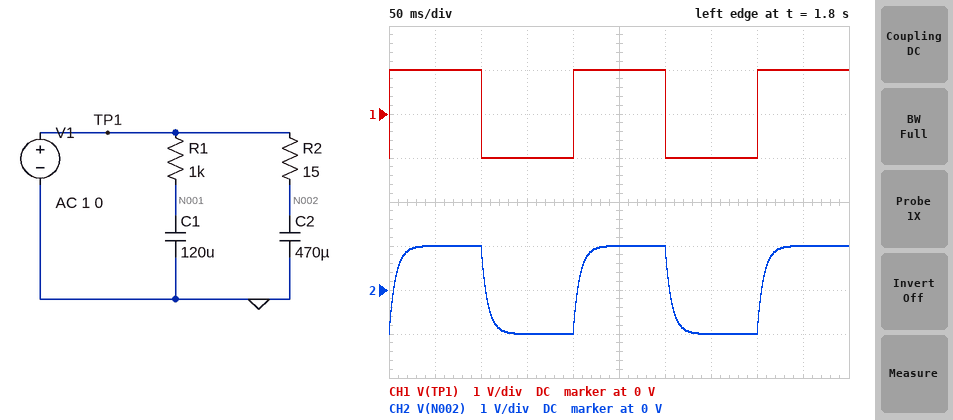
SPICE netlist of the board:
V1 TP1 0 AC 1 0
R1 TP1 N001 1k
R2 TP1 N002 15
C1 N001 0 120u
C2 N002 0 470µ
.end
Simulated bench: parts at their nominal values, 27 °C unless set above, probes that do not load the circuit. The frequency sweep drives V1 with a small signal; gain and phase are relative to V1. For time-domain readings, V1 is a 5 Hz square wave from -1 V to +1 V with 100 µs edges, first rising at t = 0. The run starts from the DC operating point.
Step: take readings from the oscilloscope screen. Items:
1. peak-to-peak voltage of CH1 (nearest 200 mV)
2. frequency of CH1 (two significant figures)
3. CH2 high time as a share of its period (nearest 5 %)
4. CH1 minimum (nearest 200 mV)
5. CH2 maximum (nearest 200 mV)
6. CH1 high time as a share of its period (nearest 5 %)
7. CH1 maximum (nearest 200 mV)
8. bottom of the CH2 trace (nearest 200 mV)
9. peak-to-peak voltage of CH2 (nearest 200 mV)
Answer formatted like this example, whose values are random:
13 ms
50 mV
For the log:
2.0 V
5.0 Hz
50 %
-1.0 V
1.0 V
50 %
1.0 V
-1.0 V
2.0 V
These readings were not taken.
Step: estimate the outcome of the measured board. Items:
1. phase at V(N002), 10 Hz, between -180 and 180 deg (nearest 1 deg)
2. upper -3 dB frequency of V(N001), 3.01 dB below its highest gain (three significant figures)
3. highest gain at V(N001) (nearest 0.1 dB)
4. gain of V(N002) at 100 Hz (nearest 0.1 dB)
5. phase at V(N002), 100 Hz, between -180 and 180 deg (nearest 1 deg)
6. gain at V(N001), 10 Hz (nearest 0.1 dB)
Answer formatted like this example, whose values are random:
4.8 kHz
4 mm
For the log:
-24 deg
1.33 Hz
0 dB
-13.1 dB
-77 deg
-17.6 dB
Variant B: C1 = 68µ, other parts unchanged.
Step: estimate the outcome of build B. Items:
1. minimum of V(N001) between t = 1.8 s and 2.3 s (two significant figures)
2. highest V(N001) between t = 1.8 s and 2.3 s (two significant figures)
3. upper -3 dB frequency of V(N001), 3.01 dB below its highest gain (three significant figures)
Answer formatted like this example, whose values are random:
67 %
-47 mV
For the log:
-630 mV
630 mV
2.34 Hz
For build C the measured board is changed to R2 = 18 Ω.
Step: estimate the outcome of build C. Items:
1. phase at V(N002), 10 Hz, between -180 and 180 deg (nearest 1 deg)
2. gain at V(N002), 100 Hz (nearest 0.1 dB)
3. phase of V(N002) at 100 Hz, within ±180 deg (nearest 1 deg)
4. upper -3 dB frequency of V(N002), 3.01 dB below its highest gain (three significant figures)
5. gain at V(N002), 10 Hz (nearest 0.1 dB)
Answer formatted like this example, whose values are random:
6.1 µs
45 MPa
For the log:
-28 deg
-14.7 dB
-79 deg
18.8 Hz
-1.1 dB
